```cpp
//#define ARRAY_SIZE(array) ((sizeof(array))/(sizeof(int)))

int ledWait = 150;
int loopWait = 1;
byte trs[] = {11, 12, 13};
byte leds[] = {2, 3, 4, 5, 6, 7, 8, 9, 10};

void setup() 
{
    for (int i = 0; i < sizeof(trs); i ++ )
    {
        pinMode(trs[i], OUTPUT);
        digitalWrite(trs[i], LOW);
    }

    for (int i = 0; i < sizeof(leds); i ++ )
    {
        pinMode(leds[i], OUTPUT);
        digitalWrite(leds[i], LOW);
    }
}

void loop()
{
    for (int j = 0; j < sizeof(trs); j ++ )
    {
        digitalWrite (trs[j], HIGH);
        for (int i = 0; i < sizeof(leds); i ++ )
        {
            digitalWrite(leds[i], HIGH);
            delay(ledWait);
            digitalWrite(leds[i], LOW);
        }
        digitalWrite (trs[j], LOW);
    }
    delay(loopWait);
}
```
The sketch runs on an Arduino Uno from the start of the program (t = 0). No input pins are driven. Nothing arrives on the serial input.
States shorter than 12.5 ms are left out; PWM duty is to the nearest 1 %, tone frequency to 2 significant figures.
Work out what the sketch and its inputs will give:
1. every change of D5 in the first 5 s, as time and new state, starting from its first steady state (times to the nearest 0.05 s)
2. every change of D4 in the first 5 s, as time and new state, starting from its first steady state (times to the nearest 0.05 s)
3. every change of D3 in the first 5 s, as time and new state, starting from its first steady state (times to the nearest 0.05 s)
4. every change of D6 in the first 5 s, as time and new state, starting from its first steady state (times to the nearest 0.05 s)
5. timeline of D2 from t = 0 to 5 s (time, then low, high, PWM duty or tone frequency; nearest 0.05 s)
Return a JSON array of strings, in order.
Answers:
["0 s low; 0.45 s high; 0.6 s low; 1.8 s high; 1.95 s low; 3.15 s high; 3.3 s low; 4.5 s high; 4.65 s low", "0 s low; 0.3 s high; 0.45 s low; 1.65 s high; 1.8 s low; 3 s high; 3.15 s low; 4.35 s high; 4.5 s low", "0 s low; 0.15 s high; 0.3 s low; 1.5 s high; 1.65 s low; 2.85 s high; 3 s low; 4.2 s high; 4.35 s low", "0 s low; 0.6 s high; 0.75 s low; 1.95 s high; 2.1 s low; 3.3 s high; 3.45 s low; 4.65 s high; 4.8 s low", "0 s high; 0.15 s low; 1.35 s high; 1.5 s low; 2.7 s high; 2.85 s low; 4.05 s high; 4.2 s low"]
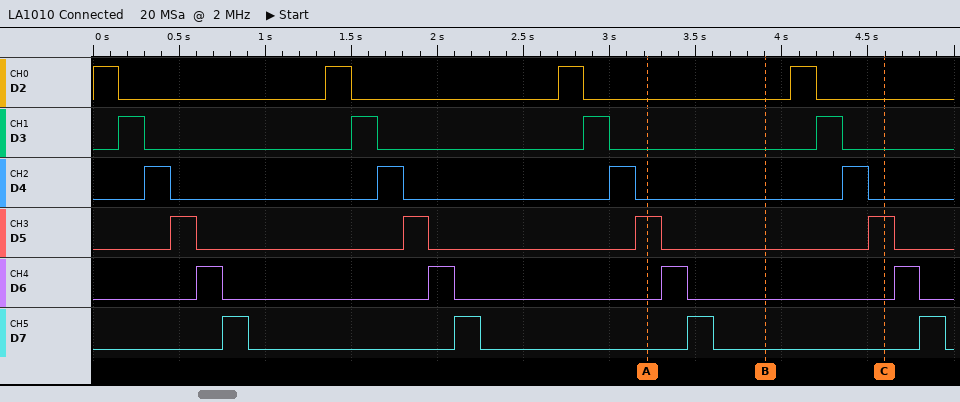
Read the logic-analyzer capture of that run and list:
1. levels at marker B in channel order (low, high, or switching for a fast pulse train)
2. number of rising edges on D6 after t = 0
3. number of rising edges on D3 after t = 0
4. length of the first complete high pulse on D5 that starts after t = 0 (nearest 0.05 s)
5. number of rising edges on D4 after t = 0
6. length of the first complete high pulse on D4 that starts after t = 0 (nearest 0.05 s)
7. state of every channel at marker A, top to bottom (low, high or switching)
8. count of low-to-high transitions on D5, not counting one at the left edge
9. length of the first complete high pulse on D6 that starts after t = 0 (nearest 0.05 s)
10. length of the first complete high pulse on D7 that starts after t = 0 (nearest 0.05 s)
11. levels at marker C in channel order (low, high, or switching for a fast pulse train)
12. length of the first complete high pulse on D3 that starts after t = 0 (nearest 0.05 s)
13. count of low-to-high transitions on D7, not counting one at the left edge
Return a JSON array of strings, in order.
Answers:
["D2 low, D3 low, D4 low, D5 low, D6 low, D7 low", "4", "4", "0.15 s", "4", "0.15 s", "D2 low, D3 low, D4 low, D5 high, D6 low, D7 low", "4", "0.15 s", "0.15 s", "D2 low, D3 low, D4 low, D5 high, D6 low, D7 low", "0.15 s", "4"]
